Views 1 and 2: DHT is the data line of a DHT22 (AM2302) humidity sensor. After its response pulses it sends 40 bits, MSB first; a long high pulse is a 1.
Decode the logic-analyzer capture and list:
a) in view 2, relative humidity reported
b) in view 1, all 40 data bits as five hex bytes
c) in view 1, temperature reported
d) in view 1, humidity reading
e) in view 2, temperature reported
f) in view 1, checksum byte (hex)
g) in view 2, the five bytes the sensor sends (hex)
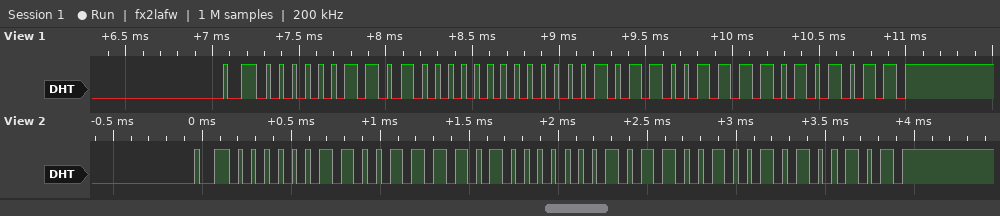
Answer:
82.9 %
03 40 01 67 AB
35.9 °C
83.2 %
35.6 °C
0xAB
03 3D 01 64 A5
